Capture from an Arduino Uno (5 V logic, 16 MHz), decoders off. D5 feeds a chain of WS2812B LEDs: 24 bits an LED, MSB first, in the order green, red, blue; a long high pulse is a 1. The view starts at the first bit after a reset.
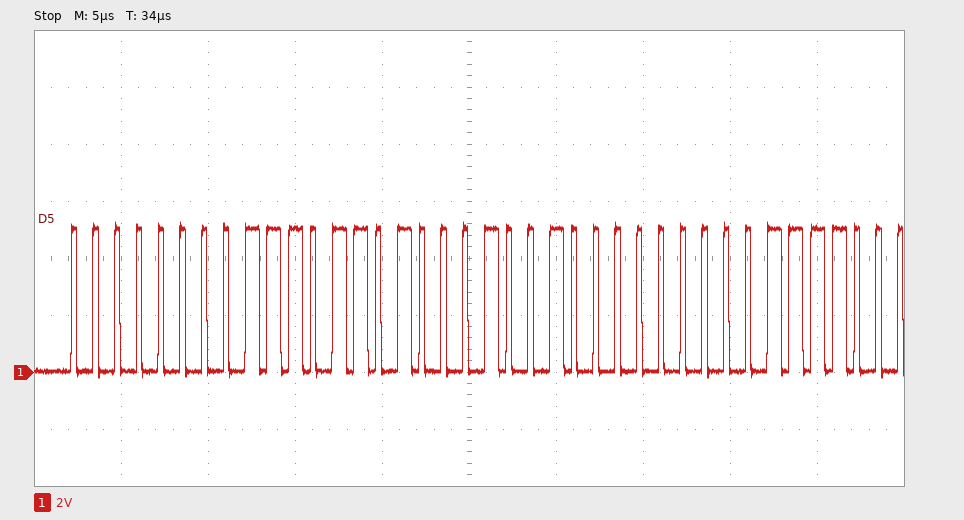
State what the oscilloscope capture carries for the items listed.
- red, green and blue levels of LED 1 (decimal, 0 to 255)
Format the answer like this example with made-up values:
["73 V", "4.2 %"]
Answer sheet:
["237, 0, 18"]
